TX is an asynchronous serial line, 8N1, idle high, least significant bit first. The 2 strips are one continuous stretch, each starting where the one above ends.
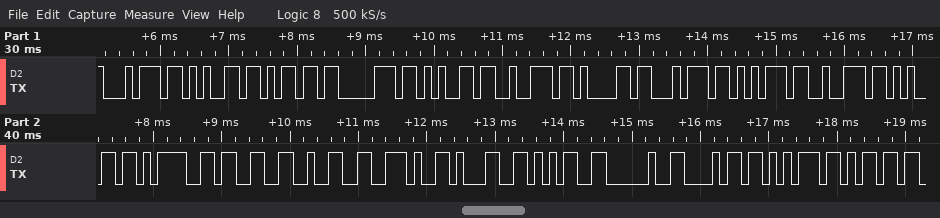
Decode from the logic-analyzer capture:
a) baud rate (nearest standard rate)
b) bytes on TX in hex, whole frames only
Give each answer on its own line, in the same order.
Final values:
9600 baud
0x74 0x65 0x6D 0x70 0x65 0x72 0x61 0x74 0x75 0x72 0x65 0x3D 0x33 0x32 0x2E 0x31 0x35 0x20 0x68 0x75 0x6D
